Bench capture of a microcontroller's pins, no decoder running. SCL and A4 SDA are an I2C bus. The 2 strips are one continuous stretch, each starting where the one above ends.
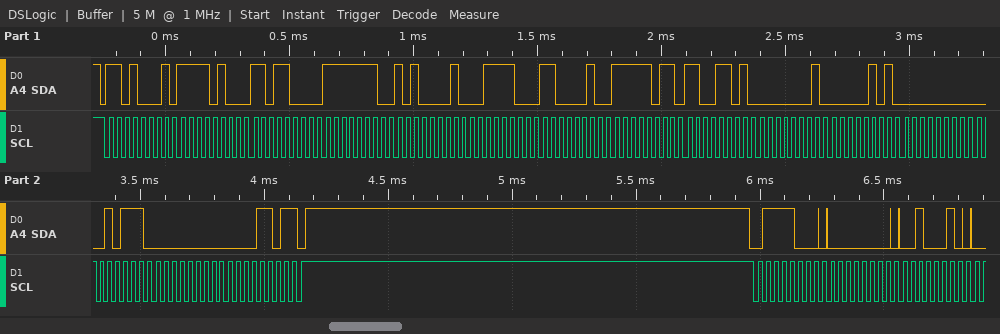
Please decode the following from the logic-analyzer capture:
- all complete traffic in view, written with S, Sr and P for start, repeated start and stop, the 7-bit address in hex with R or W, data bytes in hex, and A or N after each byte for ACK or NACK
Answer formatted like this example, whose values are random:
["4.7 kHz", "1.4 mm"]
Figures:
["S 68R A F4 A D8 A FE A A1 A 3C A C2 A FB A CD A 01 A 05 A 00 A 17 A 00 A 0D N P S 3CW A 00 A 22 A"]
